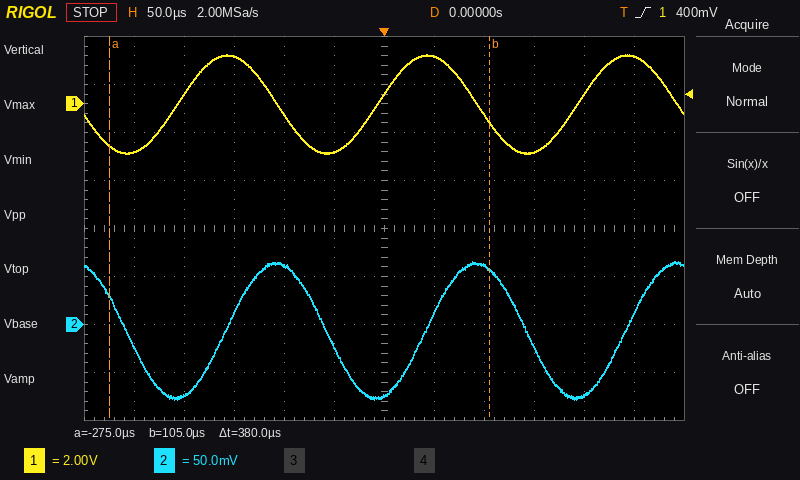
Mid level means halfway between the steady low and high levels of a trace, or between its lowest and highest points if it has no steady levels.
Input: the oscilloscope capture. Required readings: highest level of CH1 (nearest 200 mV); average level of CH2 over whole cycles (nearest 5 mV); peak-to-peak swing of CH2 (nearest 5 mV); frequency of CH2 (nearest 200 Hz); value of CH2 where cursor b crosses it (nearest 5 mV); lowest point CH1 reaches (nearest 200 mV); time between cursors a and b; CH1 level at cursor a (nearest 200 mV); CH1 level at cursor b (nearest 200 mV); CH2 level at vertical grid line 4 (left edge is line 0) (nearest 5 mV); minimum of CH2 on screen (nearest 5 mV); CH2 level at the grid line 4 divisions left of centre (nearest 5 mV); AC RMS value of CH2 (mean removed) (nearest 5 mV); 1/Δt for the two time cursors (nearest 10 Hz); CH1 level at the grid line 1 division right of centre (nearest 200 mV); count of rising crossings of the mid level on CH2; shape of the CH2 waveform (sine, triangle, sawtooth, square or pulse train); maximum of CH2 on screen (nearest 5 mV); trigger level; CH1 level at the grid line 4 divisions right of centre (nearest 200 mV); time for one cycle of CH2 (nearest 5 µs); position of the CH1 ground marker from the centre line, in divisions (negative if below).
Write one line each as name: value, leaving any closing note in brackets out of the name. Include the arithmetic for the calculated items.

highest level of CH1: 2.0 V
average level of CH2 over whole cycles: (65 mV + (-80 mV)) / 2 ≈ -7.50 mV, so -5 mV to the nearest 5 mV
peak-to-peak swing of CH2: 65 mV − (-80 mV) = 145 mV
frequency of CH2: 1 / 200 µs ≈ 5.0 kHz
value of CH2 where cursor b crosses it: 55 mV
lowest point CH1 reaches: -2.0 V
time between cursors a and b: 380 µs
CH1 level at cursor a: -1.8 V
CH1 level at cursor b: -800 mV
CH2 level at vertical grid line 4 (left edge is line 0): 60 mV
minimum of CH2 on screen: -80 mV
CH2 level at the grid line 4 divisions left of centre: -75 mV
AC RMS value of CH2 (mean removed): 145 mV / (2√2) ≈ 51.3 mV, so 50 mV to the nearest 5 mV
1/Δt for the two time cursors: 1 / 380 µs ≈ 2.63 kHz
CH1 level at the grid line 1 division right of centre: 2.0 V
count of rising crossings of the mid level on CH2: 3
shape of the CH2 waveform: sine
maximum of CH2 on screen: 65 mV
trigger level: 400 mV
CH1 level at the grid line 4 divisions right of centre: 400 mV
time for one cycle of CH2: 200 µs
position of the CH1 ground marker from the centre line, in divisions: +2.6 div
